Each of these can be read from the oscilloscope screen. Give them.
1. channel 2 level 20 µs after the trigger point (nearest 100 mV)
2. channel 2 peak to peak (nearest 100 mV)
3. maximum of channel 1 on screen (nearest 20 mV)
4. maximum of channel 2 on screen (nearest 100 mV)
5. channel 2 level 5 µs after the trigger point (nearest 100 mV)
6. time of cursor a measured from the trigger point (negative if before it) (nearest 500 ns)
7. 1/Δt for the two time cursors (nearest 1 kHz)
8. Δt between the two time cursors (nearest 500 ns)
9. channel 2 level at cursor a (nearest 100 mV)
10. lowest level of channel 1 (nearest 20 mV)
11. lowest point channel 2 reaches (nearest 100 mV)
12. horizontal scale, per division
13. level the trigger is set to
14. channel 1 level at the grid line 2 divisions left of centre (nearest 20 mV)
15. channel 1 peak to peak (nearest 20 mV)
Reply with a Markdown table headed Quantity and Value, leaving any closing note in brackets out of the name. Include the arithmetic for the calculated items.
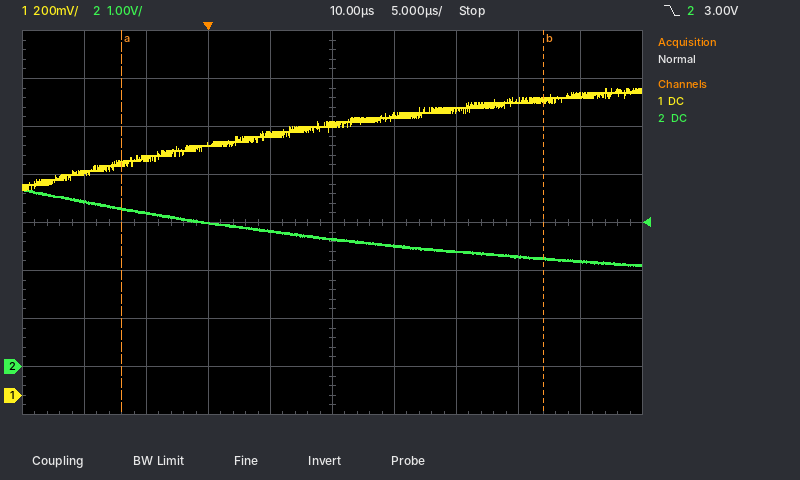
| Quantity | Value |
|---|---|
| channel 2 level 20 µs after the trigger point | 2.4 V |
| channel 2 peak to peak | 3.7 V − (2.1 V) = 1.6 V |
| maximum of channel 1 on screen | 1.28 V |
| maximum of channel 2 on screen | 3.7 V |
| channel 2 level 5 µs after the trigger point | 2.8 V |
| time of cursor a measured from the trigger point (negative if before it) | -7.0 µs |
| 1/Δt for the two time cursors | 1 / 34.0 µs ≈ 29 kHz |
| Δt between the two time cursors | 34.0 µs |
| channel 2 level at cursor a | 3.3 V |
| lowest level of channel 1 | 860 mV |
| lowest point channel 2 reaches | 2.1 V |
| horizontal scale, per division | 5 µs |
| level the trigger is set to | 3.00 V |
| channel 1 level at the grid line 2 divisions left of centre | 1.04 V |
| channel 1 peak to peak | 1.28 V − (860 mV) = 420 mV |
